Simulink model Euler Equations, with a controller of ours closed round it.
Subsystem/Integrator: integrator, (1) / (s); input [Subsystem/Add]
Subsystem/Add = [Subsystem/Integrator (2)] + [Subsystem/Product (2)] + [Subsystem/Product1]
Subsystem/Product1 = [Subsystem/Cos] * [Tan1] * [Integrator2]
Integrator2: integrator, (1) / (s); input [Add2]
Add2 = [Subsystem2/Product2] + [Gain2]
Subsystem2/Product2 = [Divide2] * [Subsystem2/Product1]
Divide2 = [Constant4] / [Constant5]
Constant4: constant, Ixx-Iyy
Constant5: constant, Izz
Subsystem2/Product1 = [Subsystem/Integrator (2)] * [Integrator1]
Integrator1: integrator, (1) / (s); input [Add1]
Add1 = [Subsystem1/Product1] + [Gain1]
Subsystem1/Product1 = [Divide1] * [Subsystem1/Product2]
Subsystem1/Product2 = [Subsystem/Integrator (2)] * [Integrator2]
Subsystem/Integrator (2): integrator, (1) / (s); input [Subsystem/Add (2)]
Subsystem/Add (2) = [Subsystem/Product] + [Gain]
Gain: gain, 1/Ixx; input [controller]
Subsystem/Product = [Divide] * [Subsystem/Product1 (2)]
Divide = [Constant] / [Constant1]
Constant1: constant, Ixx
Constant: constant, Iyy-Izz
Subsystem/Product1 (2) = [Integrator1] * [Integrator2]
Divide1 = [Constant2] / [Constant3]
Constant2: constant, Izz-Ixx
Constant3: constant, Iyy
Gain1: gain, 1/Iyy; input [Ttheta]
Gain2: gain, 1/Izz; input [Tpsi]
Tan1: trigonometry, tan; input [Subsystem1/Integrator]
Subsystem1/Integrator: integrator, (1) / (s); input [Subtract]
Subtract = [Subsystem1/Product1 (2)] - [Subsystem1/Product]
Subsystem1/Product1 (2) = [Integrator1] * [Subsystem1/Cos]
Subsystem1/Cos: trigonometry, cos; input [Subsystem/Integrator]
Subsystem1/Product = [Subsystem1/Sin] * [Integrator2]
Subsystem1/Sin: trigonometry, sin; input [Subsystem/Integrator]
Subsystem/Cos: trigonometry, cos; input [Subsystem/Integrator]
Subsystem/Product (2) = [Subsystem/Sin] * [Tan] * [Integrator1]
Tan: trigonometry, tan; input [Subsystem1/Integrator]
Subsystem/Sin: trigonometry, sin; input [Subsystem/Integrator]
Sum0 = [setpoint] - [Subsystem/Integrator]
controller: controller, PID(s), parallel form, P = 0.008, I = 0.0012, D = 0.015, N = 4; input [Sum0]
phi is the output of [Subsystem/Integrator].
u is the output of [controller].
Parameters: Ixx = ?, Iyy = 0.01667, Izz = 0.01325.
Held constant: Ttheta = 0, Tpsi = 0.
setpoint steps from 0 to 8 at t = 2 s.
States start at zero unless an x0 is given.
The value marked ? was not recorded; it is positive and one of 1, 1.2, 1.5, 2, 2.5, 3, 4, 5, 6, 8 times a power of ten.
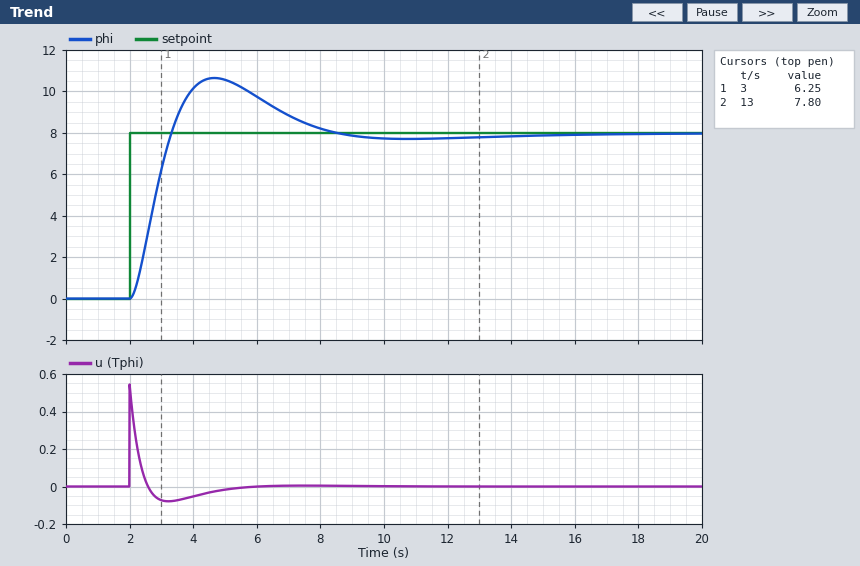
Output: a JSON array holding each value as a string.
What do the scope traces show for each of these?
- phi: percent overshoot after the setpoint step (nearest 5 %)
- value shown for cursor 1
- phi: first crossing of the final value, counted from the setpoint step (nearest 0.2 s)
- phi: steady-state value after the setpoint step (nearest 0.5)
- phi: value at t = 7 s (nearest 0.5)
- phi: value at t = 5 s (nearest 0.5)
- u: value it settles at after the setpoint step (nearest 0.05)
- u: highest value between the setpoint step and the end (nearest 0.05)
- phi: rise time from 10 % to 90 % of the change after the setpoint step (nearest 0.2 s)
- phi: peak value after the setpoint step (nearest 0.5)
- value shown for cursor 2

["35 %", "6.25", "1.4 s", "8.0", "9.0", "10.5", "0.00", "0.55", "1.0 s", "10.5", "7.80"]
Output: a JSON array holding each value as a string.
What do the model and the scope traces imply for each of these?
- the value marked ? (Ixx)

["0.015"]
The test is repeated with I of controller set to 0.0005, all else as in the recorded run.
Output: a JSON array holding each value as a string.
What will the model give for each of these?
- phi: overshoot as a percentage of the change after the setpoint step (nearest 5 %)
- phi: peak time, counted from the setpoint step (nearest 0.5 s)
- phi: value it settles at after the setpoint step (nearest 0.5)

["30 %", "2.5 s", "8.0"]
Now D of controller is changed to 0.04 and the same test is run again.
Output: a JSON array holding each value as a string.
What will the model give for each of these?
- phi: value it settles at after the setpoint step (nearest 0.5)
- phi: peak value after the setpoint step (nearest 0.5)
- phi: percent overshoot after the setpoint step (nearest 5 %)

["8.0", "9.5", "20 %"]
